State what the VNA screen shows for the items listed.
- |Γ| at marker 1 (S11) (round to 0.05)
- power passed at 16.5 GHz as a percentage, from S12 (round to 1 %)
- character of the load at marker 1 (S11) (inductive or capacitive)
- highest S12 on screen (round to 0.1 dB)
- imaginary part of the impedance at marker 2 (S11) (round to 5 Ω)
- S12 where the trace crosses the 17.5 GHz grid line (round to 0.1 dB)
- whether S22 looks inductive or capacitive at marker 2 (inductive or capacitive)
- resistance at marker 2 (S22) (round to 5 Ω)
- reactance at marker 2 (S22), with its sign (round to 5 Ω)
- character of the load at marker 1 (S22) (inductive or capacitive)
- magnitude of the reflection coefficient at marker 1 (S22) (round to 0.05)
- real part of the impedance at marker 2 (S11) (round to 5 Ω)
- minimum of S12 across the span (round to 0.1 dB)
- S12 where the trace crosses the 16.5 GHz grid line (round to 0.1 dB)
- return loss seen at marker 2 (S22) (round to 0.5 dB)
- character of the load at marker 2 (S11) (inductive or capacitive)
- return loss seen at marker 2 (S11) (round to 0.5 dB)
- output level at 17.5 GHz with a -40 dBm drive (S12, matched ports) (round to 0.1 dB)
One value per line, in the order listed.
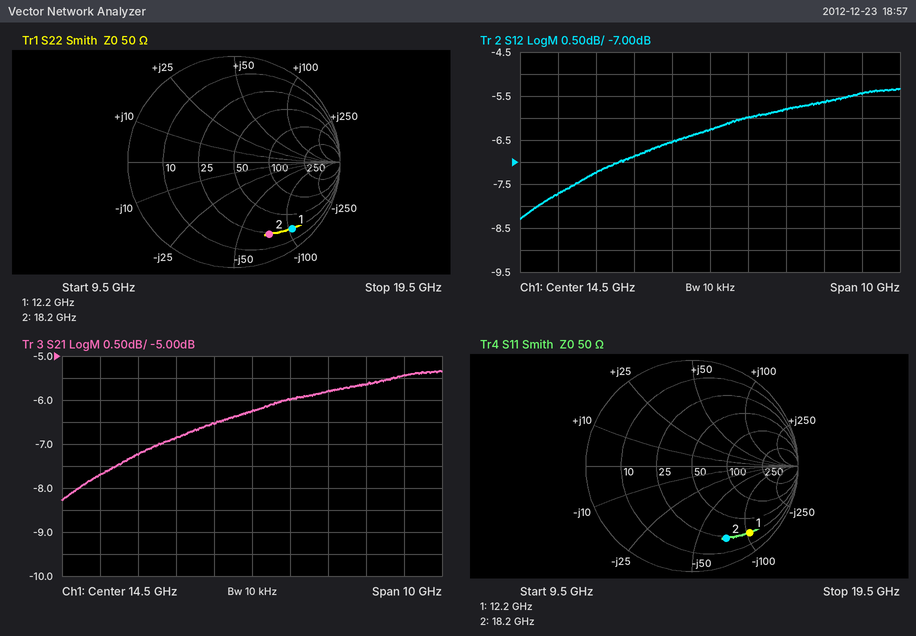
0.85
26 %
capacitive
-5.3 dB
-75 Ω
-5.6 dB
capacitive
25 Ω
-75 Ω
capacitive
0.85
25 Ω
-8.3 dB
-5.8 dB
2.5 dB
capacitive
2.5 dB
-45.6 dBm
